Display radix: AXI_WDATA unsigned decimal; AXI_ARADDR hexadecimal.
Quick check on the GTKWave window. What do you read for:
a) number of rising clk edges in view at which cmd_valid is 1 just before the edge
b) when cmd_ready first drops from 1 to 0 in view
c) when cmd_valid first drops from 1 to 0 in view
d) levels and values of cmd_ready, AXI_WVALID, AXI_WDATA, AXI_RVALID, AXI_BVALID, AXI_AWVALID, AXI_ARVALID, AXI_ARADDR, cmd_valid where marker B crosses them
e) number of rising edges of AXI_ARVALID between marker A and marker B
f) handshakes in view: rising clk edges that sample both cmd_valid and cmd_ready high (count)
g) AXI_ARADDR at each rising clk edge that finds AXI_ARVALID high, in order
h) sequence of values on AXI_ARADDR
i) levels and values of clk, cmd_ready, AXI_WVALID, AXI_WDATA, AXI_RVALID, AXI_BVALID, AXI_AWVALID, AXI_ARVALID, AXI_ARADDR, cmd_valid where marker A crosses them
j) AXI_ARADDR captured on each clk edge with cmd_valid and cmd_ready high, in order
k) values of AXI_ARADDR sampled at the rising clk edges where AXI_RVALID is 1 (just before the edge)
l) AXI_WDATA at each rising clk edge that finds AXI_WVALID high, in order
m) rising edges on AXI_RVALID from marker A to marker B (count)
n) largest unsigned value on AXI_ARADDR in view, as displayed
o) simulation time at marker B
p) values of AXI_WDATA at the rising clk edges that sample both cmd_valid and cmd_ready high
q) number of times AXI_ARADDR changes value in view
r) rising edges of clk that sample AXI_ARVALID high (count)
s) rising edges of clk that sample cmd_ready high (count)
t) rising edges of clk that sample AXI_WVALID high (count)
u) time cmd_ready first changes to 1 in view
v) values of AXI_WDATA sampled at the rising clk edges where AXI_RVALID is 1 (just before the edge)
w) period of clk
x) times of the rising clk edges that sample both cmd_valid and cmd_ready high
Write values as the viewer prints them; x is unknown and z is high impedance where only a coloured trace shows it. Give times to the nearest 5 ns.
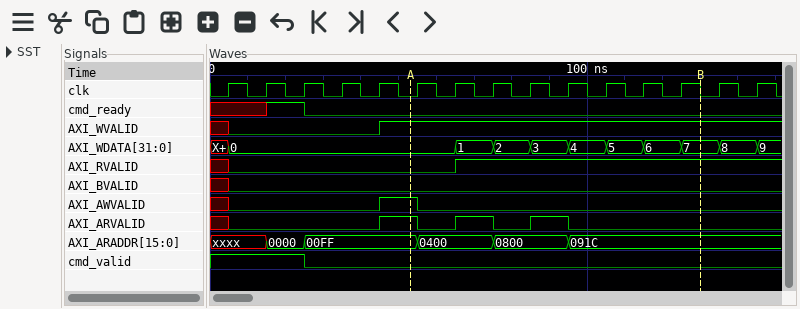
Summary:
3
25 ns
25 ns
cmd_ready=0, AXI_WVALID=1, AXI_WDATA=7, AXI_RVALID=1, AXI_BVALID=0, AXI_AWVALID=0, AXI_ARVALID=0, AXI_ARADDR=091C, cmd_valid=0
2
1
00FF, 0400, 0800
xxxx, 0000, 00FF, 0400, 0800, 091C
clk=0, cmd_ready=0, AXI_WVALID=1, AXI_WDATA=0, AXI_RVALID=0, AXI_BVALID=0, AXI_AWVALID=1, AXI_ARVALID=1, AXI_ARADDR=00FF, cmd_valid=0
0000
0400, 0800, 0800, 091C, 091C, 091C, 091C, 091C
0, 0, 1, 2, 3, 4, 5, 6, 7, 8
1
091C
130 ns
0
5
3
1
10
15 ns
1, 2, 3, 4, 5, 6, 7, 8
10 ns
25 ns
